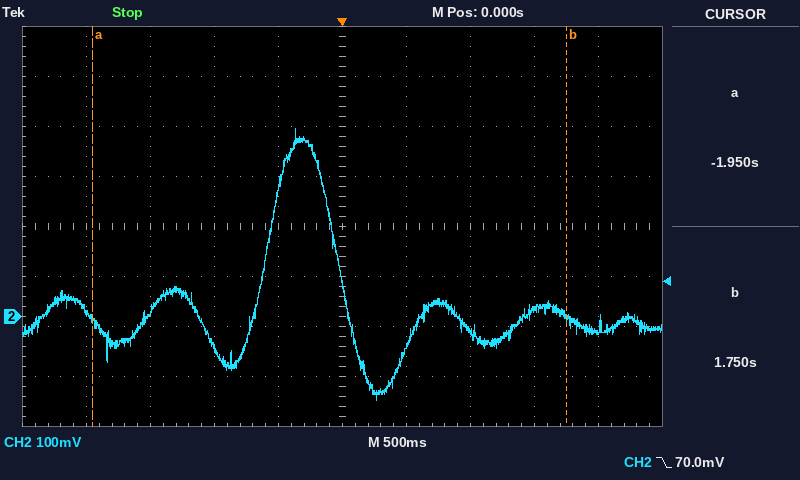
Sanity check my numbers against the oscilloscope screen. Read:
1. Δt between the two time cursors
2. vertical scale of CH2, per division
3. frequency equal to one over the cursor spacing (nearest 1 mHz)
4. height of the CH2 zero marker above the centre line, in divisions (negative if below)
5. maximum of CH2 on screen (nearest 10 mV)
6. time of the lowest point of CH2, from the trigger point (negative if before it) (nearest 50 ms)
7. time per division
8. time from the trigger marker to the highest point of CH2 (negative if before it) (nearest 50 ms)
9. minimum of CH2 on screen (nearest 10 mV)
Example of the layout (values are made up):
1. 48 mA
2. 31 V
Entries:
1. 3.70 s
2. 100 mV
3. 270 mHz
4. -1.8 div
5. 380 mV
6. +250 ms
7. 500 ms
8. -350 ms
9. -170 mV
